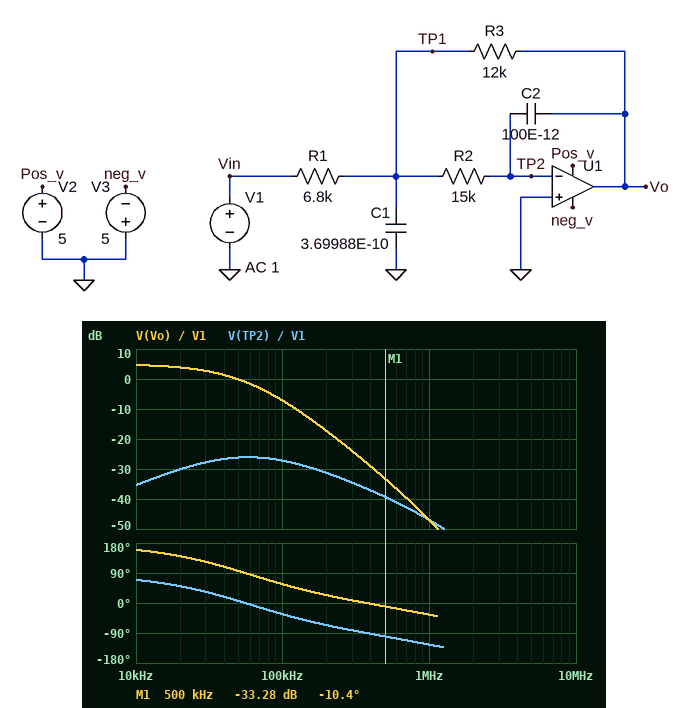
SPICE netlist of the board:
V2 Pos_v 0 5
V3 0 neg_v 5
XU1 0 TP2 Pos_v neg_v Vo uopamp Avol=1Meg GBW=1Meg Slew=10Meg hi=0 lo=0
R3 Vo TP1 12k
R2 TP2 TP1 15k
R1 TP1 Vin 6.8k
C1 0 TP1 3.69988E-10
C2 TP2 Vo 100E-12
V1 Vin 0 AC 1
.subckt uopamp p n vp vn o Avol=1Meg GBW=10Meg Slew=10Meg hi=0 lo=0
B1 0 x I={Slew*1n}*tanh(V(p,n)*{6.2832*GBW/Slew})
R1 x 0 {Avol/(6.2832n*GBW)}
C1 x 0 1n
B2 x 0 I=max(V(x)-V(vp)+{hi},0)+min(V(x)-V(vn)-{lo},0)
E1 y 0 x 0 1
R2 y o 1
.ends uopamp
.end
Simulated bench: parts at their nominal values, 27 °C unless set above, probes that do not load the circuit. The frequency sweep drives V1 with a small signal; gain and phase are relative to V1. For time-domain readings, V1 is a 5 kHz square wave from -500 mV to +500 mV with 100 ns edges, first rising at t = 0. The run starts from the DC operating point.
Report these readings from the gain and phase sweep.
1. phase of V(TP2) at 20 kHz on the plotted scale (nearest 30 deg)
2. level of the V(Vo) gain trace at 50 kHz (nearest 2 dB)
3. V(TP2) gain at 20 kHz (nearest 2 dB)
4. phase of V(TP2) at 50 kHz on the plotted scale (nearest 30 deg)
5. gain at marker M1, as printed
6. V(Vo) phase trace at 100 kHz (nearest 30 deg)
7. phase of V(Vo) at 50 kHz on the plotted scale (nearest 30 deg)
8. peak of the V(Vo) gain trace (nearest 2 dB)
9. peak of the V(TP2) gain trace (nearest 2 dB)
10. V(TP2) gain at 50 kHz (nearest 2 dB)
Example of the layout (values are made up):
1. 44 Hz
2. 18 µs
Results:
1. 60 deg
2. 0 dB
3. -30 dB
4. 0 deg
5. -33.28 dB
6. 60 deg
7. 90 deg
8. 4 dB
9. -26 dB
10. -26 dB
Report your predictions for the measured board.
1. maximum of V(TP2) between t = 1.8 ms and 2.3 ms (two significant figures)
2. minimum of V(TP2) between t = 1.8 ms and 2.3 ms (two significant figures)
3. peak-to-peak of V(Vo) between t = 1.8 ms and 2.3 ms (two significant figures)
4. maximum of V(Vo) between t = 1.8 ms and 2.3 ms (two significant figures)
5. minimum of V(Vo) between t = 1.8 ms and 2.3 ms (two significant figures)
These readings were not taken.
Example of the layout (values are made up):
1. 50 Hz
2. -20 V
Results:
1. 37 mV
2. -37 mV
3. 1.8 V
4. 880 mV
5. -880 mV
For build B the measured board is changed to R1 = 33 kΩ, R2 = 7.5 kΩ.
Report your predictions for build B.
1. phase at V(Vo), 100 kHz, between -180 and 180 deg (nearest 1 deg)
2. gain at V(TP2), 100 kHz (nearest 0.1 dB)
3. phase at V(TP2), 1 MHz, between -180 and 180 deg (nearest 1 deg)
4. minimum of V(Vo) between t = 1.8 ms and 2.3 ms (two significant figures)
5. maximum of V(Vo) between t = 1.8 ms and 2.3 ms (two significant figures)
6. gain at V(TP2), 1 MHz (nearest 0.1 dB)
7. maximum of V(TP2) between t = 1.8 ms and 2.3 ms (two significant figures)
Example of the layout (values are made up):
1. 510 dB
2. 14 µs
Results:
1. 62 deg
2. -32.8 dB
3. -124 deg
4. -220 mV
5. 220 mV
6. -55.1 dB
7. 15 mV
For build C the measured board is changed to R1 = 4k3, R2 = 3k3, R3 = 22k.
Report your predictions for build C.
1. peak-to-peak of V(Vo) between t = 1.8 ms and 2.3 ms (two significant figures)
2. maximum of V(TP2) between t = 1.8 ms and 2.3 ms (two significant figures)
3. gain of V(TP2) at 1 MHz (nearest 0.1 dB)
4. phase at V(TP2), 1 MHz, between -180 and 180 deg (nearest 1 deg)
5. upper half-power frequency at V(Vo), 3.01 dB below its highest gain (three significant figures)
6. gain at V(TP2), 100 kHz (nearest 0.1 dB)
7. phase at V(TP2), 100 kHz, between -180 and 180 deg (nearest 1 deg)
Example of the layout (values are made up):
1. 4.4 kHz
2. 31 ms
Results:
1. 5.1 V
2. 130 mV
3. -31.7 dB
4. -112 deg
5. 36.9 kHz
6. -16.1 dB
7. -15 deg
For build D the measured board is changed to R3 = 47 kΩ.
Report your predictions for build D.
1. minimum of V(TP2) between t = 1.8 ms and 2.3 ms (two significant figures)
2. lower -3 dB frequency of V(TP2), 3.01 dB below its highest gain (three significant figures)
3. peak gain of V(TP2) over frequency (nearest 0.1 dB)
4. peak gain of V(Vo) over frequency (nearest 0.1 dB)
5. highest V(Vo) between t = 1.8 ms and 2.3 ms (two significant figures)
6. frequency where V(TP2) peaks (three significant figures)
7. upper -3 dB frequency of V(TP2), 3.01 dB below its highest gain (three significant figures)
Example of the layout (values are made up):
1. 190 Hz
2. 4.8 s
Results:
1. -52 mV
2. 8.29 kHz
3. -24.1 dB
4. 16.8 dB
5. 3.4 V
6. 29.5 kHz
7. 105 kHz
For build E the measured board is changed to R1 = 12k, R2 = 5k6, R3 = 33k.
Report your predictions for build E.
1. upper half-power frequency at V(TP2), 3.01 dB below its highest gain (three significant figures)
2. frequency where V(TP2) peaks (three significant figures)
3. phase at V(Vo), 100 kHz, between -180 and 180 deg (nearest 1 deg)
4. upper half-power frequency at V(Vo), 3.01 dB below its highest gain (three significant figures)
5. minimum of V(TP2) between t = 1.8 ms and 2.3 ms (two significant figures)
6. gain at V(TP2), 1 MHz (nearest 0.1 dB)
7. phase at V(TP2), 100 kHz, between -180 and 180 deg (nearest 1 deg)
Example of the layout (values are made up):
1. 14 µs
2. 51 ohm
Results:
1. 126 kHz
2. 53.2 kHz
3. 51 deg
4. 35.1 kHz
5. -55 mV
6. -44.2 dB
7. -39 deg
